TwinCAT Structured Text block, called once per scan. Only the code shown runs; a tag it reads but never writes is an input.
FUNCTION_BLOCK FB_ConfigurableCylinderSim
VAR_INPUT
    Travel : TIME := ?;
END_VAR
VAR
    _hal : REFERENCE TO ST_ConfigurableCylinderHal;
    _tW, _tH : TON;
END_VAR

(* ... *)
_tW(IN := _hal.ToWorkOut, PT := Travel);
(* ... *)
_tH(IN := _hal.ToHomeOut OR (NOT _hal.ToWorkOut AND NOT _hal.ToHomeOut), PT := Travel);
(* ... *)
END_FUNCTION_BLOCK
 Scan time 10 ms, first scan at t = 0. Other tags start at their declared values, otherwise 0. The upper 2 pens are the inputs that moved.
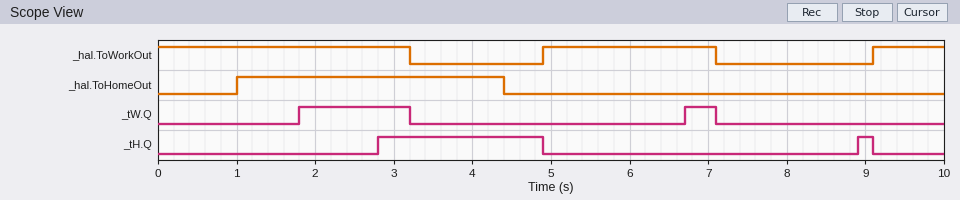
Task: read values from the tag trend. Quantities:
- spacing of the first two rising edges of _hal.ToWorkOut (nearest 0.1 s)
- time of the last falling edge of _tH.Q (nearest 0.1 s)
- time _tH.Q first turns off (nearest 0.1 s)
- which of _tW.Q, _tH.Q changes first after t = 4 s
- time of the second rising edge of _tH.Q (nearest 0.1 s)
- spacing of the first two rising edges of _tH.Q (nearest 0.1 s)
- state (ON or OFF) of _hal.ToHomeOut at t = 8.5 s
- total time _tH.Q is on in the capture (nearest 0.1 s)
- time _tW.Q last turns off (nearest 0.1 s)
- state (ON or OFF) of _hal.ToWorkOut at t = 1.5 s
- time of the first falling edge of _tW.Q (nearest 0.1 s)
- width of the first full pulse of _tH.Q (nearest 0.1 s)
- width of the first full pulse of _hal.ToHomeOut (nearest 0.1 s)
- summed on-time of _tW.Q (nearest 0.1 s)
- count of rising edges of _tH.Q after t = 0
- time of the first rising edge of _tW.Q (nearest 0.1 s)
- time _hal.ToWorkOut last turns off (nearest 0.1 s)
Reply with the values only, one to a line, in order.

4.2 s
9.1 s
4.9 s
_tH.Q
8.9 s
6.1 s
OFF
2.3 s
7.1 s
ON
3.2 s
2.1 s
3.4 s
1.8 s
2
1.8 s
7.1 s
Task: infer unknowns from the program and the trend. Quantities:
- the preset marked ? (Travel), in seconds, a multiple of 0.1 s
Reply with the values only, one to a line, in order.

1.8 s
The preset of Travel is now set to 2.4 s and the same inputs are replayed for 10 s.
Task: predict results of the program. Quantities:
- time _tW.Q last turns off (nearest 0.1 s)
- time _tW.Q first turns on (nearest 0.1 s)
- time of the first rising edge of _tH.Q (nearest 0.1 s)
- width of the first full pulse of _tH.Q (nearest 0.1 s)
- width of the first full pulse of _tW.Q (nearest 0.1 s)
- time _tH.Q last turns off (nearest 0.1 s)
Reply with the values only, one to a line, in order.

3.2 s
2.4 s
3.4 s
1.5 s
0.8 s
4.9 s
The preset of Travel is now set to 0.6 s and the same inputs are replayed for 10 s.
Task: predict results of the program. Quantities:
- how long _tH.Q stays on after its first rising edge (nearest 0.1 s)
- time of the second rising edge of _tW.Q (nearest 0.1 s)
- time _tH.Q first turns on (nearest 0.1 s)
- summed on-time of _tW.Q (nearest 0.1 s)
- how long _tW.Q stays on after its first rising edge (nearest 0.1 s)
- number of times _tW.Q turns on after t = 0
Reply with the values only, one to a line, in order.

3.3 s
5.5 s
1.6 s
4.5 s
2.6 s
3
